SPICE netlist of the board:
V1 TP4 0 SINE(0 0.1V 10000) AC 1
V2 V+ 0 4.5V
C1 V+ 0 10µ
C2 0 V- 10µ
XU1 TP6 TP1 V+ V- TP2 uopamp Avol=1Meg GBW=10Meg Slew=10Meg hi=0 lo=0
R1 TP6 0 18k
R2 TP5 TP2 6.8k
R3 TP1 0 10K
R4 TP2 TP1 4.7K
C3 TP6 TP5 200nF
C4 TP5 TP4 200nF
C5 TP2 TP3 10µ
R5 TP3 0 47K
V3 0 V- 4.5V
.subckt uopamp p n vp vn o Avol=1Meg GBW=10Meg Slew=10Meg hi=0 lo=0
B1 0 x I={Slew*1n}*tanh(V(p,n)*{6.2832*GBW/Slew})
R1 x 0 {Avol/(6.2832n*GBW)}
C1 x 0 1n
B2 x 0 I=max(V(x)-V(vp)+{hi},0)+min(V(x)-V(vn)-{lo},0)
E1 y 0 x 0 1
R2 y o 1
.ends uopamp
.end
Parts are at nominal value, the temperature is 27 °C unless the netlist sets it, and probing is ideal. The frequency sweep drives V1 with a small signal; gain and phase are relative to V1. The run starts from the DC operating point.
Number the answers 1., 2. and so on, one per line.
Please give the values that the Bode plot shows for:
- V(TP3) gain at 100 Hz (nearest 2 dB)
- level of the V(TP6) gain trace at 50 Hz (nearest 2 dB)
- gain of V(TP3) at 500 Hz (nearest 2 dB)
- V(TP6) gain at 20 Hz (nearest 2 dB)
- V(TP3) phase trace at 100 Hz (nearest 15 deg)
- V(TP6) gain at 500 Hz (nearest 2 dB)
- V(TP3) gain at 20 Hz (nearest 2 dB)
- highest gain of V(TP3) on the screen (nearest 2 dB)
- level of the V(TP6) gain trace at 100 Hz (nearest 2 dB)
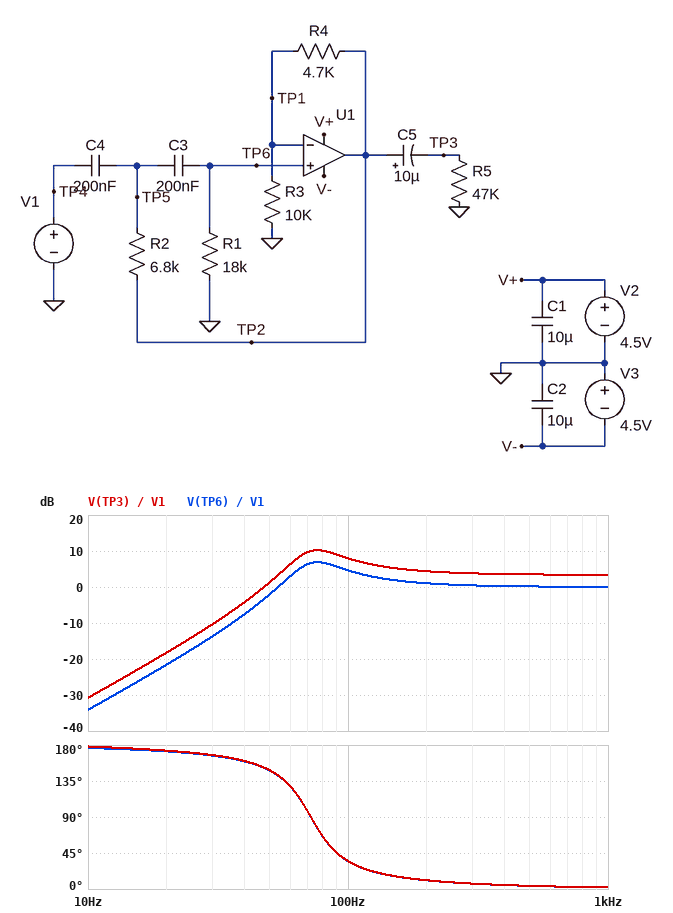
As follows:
1. 8 dB
2. -2 dB
3. 4 dB
4. -22 dB
5. 30 deg
6. 0 dB
7. -18 dB
8. 10 dB
9. 4 dB
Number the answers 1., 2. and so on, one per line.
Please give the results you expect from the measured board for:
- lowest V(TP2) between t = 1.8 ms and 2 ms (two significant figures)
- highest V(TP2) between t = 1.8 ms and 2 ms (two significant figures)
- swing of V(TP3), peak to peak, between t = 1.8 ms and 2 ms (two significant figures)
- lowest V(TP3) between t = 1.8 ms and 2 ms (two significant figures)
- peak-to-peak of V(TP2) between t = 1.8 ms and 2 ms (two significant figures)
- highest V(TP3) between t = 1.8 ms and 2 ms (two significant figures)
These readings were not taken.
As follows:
1. -150 mV
2. 150 mV
3. 290 mV
4. -150 mV
5. 290 mV
6. 150 mV
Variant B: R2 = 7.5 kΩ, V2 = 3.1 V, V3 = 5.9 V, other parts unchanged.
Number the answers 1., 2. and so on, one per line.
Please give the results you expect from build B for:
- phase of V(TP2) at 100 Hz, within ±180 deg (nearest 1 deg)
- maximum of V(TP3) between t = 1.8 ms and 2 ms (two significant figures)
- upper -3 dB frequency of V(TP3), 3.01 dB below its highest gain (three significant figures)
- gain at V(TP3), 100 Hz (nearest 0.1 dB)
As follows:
1. 36 deg
2. 150 mV
3. 125 Hz
4. 7.0 dB
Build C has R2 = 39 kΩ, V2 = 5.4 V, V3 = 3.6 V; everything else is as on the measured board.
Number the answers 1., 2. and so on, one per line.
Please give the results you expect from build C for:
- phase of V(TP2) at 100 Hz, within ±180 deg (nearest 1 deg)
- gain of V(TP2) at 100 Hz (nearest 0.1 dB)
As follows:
1. 41 deg
2. 1.7 dB
